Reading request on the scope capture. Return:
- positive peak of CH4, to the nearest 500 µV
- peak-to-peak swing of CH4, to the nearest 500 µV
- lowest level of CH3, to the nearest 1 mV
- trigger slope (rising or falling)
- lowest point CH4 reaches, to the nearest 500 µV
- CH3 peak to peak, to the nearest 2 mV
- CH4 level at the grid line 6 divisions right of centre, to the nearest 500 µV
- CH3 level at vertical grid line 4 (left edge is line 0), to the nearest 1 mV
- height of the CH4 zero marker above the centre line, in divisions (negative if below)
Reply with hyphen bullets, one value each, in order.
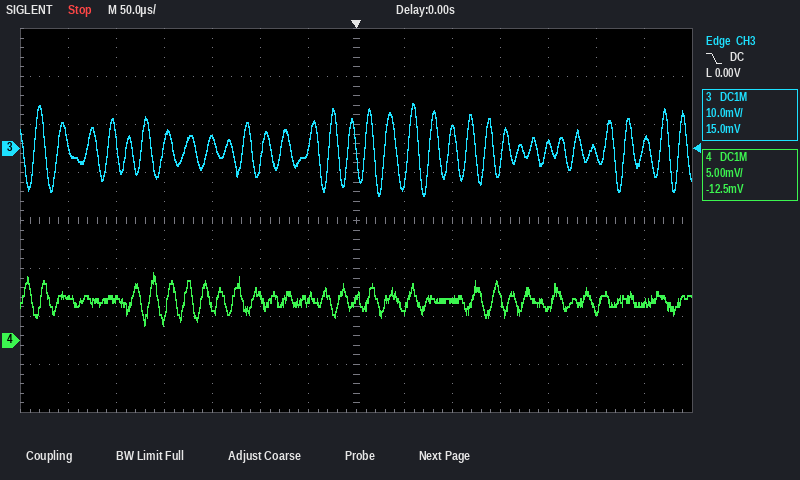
- 7.0 mV
- 5.5 mV
- -10 mV
- falling
- 1.5 mV
- 20 mV
- 4.0 mV
- 2 mV
- -2.5 div
